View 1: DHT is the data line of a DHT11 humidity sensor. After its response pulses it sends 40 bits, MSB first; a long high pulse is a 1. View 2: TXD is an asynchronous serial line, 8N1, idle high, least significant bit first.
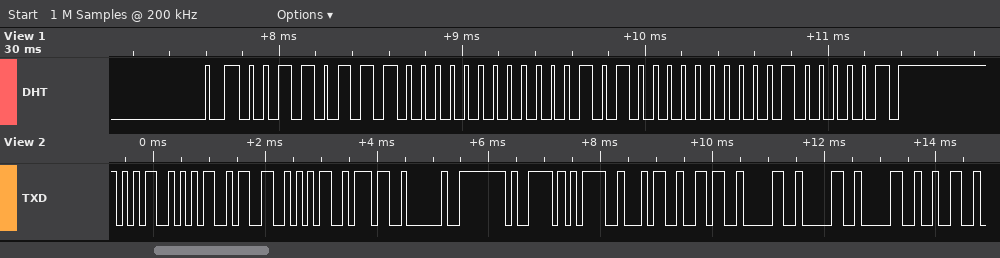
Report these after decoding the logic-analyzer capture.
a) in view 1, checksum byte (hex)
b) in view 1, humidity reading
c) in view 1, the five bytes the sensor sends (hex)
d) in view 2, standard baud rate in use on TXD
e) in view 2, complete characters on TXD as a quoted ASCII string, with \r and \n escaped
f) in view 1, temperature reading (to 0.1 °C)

0x41
55 %
37 00 0A 00 41
9600 baud
"55357 y=460002"
10.0 °C
